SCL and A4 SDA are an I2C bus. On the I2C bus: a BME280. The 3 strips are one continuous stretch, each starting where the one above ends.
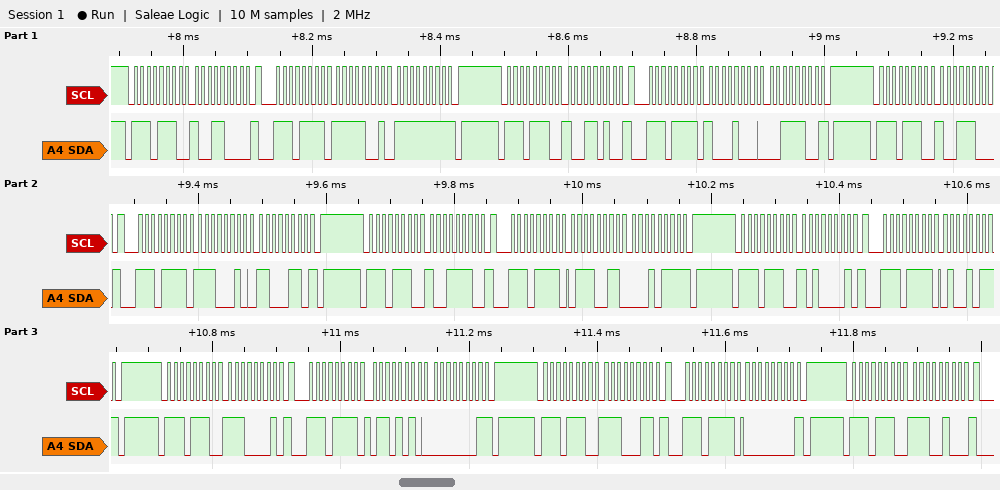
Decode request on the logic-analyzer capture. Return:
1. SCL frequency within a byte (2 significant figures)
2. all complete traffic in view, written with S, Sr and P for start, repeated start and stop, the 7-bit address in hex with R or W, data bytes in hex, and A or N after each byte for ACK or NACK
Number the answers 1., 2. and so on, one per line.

1. 100 kHz
2. S 77W A 98 A Sr 77R A F9 A FF N P S 77W A 9A A Sr 77R A 88 A 3C N P S 77W A 9C A Sr 77R A E2 A C6 N P S 77W A 9E A Sr 77R A 73 A 17 N P S 77W A A1 A Sr 77R A 4B N P S 77W A E1 A Sr 77R A 6A A 01 N P S 77W A E3 A Sr 77R A 00 N P S 77W A E4 A
